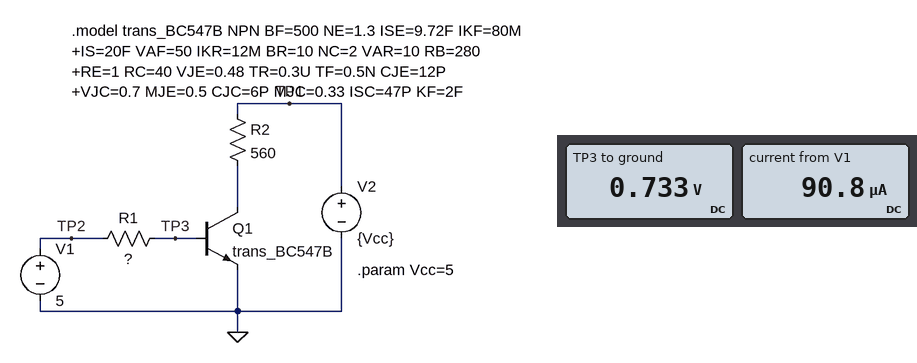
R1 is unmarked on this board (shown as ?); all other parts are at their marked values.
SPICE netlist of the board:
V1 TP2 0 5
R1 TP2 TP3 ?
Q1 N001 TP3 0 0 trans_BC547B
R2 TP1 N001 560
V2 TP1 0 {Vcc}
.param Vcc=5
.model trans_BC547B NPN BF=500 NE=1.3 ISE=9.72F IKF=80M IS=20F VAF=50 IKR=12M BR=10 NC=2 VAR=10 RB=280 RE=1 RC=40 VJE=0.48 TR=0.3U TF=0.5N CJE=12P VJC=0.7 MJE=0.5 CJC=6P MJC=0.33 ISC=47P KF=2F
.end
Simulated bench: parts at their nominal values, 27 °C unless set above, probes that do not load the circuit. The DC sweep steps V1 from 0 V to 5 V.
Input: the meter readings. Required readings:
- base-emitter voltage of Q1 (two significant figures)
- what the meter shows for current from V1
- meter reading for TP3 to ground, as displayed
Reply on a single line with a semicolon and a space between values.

730 mV; 90.8 µA; 0.733 V
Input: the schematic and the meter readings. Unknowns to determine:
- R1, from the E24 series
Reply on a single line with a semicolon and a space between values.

47 kΩ
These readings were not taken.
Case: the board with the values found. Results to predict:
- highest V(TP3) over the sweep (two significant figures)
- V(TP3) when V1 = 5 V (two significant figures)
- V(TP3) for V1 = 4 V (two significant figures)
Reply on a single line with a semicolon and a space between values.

730 mV; 730 mV; 730 mV
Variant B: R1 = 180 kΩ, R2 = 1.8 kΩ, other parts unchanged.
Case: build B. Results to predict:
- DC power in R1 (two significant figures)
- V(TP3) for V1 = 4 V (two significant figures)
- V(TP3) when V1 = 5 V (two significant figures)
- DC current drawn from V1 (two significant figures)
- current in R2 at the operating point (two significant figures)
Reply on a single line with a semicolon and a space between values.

100 µW; 670 mV; 680 mV; 24 µA; 2.7 mA
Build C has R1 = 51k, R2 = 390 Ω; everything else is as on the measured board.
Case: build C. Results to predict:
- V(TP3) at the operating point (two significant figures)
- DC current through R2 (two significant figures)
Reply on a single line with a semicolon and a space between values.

740 mV; 11 mA
